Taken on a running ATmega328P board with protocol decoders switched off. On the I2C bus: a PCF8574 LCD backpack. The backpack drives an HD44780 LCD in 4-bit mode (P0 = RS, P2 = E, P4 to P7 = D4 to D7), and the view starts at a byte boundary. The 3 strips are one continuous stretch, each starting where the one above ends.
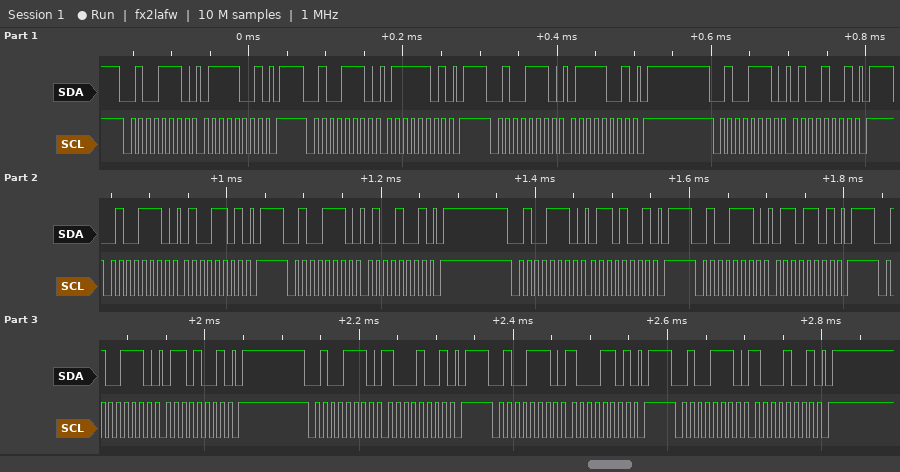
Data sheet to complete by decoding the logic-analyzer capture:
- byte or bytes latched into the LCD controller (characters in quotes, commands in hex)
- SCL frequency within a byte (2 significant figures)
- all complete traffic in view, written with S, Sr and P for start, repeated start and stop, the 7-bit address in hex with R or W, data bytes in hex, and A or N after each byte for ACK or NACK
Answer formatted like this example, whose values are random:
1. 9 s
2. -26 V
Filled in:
1. 't' 'h'
2. 100 kHz
3. S 27W A 79 A P S 27W A 7D A P S 27W A 79 A P S 27W A 49 A P S 27W A 4D A P S 27W A 49 A P S 27W A 69 A P S 27W A 6D A P S 27W A 69 A P S 27W A 89 A P S 27W A 8D A P S 27W A 89 A P
